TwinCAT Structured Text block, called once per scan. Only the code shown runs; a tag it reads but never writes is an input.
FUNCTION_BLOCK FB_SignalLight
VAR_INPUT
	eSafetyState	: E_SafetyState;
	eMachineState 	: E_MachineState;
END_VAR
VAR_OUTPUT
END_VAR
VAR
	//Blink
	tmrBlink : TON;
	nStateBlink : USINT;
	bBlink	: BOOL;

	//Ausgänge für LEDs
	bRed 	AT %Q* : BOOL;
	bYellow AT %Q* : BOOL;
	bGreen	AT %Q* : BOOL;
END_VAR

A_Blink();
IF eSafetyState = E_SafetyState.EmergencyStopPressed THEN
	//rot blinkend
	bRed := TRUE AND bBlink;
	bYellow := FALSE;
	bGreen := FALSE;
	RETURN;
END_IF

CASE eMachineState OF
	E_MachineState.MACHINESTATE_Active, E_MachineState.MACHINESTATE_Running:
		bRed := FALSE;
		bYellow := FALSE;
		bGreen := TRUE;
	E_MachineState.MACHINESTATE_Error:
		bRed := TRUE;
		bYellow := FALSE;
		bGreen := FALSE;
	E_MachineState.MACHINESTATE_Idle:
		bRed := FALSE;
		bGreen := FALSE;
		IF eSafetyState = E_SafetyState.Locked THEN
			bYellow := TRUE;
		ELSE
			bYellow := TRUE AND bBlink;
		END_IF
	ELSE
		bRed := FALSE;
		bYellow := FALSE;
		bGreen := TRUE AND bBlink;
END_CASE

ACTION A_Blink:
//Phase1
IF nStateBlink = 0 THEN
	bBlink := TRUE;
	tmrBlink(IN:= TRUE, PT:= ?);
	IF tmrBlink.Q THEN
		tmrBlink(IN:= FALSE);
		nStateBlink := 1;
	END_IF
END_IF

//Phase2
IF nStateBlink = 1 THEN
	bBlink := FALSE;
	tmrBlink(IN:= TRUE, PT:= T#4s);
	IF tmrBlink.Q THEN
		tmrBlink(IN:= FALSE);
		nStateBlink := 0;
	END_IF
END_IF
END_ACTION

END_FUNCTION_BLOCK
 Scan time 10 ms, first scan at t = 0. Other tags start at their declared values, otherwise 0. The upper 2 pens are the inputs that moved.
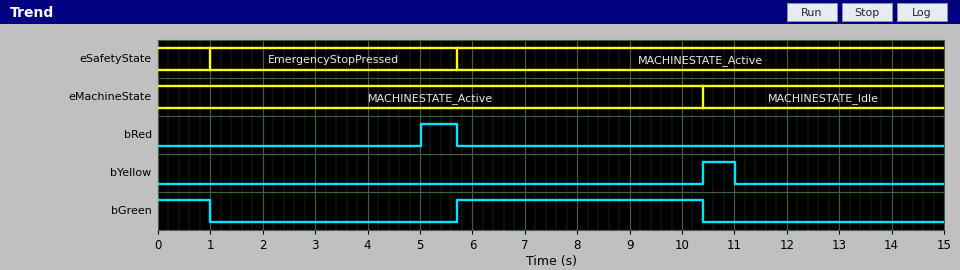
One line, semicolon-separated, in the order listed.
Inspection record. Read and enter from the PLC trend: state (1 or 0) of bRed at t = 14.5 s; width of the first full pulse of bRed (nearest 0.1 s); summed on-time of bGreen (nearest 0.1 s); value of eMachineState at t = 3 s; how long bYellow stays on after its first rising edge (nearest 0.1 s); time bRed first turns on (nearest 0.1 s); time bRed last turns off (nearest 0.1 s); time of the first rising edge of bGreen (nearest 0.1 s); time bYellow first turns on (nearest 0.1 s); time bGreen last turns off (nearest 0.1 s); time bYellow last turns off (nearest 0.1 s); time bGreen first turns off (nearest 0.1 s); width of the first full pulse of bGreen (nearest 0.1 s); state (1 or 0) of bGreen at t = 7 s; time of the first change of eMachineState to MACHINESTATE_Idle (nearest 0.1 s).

0; 0.7 s; 5.7 s; MACHINESTATE_Active; 0.6 s; 5.0 s; 5.7 s; 5.7 s; 10.4 s; 10.4 s; 11.0 s; 1.0 s; 4.7 s; 1; 10.4 s
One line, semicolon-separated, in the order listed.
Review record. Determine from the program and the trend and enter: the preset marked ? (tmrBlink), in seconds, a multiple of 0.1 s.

1.0 s
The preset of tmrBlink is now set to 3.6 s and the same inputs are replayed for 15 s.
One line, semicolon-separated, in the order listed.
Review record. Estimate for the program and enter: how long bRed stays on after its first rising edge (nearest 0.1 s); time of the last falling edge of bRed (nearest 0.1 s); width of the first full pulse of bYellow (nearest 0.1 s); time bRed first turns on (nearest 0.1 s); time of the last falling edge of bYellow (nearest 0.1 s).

2.6 s; 3.6 s; 0.8 s; 1.0 s; 11.2 s
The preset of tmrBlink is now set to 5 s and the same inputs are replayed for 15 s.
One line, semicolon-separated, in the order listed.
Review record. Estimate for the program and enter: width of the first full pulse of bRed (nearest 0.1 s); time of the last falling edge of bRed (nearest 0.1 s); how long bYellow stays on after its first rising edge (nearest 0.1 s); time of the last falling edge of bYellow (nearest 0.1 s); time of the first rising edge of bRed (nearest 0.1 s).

4.0 s; 5.0 s; 3.6 s; 14.0 s; 1.0 s
